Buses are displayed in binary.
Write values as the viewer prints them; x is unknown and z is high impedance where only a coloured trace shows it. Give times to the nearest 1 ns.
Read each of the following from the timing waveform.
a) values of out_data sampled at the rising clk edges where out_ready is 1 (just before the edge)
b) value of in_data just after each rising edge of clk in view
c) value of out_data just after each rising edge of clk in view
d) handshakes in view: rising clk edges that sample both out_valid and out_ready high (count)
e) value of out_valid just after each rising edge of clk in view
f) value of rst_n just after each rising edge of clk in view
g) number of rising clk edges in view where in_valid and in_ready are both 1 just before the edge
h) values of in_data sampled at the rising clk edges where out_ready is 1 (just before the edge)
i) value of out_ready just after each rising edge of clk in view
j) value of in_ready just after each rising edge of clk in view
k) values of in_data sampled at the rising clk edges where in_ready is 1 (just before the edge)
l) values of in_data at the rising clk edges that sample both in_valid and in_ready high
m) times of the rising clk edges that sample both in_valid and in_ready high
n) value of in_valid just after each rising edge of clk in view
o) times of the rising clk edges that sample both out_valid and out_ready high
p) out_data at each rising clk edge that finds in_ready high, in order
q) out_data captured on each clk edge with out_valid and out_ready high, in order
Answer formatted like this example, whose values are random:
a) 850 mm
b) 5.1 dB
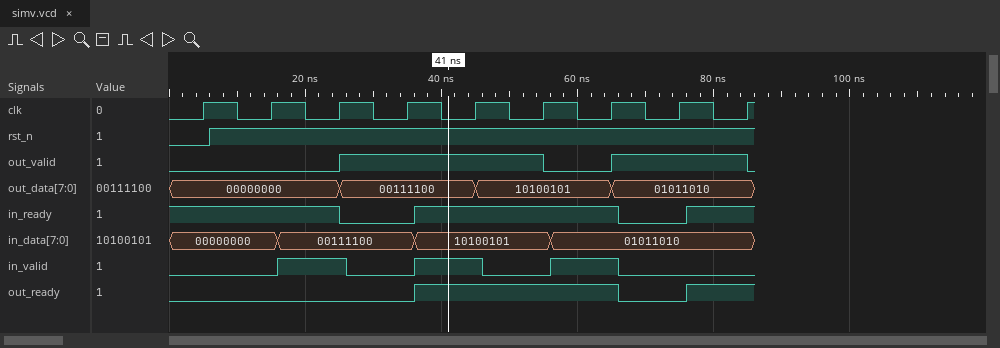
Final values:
a) 00111100, 10100101, 10100101, 01011010
b) 00000000, 00000000, 00111100, 00111100, 10100101, 10100101, 01011010, 01011010, 01011010
c) 00000000, 00000000, 00111100, 00111100, 10100101, 10100101, 01011010, 01011010, 01011010
d) 3
e) 0 0 1 1 1 0 1 1 0
f) 0 1 1 1 1 1 1 1 1
g) 3
h) 10100101, 10100101, 01011010, 01011010
i) 0 0 0 0 1 1 1 0 1
j) 1 1 0 0 1 1 1 0 1
k) 00000000, 00000000, 00111100, 10100101, 10100101, 01011010, 01011010
l) 00111100, 10100101, 01011010
m) 25 ns, 45 ns, 65 ns
n) 0 0 1 0 1 0 1 0 0
o) 45 ns, 55 ns, 85 ns
p) 00000000, 00000000, 00000000, 00111100, 10100101, 10100101, 01011010
q) 00111100, 10100101, 01011010
